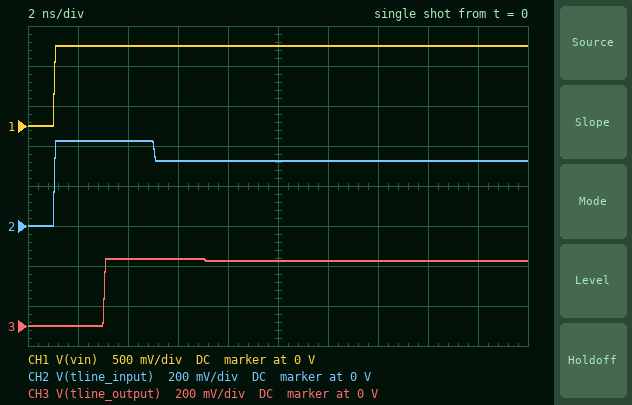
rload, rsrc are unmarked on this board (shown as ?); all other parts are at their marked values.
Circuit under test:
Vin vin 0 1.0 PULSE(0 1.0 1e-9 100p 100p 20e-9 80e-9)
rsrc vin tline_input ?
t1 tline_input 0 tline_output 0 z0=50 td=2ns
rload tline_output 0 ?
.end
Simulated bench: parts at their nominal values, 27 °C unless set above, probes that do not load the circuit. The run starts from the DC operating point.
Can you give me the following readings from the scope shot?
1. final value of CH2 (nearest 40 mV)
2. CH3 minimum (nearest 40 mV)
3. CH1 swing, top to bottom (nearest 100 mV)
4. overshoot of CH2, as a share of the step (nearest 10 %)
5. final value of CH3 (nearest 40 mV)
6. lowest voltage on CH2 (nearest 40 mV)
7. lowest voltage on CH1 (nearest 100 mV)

320 mV
0 V
1.0 V
30 %
320 mV
0 V
0 V
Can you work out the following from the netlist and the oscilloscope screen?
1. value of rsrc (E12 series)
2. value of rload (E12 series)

68 Ω
33 Ω
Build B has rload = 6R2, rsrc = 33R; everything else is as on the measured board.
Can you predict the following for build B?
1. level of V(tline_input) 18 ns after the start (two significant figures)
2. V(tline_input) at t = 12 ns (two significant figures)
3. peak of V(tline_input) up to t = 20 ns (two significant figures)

160 mV
170 mV
600 mV
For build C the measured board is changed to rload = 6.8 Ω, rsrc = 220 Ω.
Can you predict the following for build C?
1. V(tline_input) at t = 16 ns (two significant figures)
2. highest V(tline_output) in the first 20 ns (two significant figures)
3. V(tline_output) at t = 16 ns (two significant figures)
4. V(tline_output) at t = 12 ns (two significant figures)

13 mV
44 mV
28 mV
33 mV
